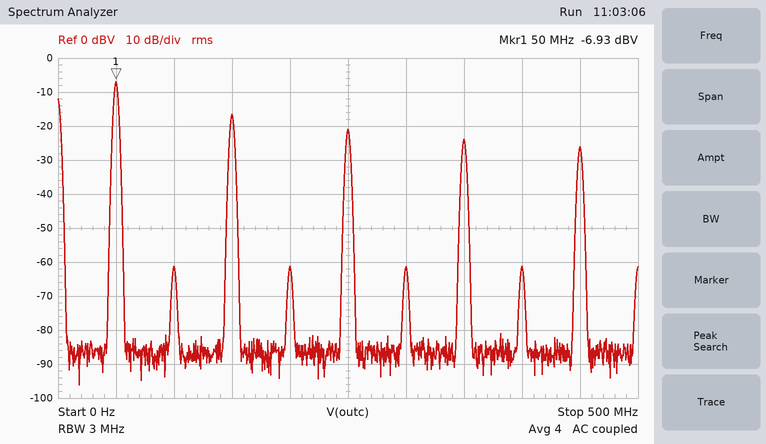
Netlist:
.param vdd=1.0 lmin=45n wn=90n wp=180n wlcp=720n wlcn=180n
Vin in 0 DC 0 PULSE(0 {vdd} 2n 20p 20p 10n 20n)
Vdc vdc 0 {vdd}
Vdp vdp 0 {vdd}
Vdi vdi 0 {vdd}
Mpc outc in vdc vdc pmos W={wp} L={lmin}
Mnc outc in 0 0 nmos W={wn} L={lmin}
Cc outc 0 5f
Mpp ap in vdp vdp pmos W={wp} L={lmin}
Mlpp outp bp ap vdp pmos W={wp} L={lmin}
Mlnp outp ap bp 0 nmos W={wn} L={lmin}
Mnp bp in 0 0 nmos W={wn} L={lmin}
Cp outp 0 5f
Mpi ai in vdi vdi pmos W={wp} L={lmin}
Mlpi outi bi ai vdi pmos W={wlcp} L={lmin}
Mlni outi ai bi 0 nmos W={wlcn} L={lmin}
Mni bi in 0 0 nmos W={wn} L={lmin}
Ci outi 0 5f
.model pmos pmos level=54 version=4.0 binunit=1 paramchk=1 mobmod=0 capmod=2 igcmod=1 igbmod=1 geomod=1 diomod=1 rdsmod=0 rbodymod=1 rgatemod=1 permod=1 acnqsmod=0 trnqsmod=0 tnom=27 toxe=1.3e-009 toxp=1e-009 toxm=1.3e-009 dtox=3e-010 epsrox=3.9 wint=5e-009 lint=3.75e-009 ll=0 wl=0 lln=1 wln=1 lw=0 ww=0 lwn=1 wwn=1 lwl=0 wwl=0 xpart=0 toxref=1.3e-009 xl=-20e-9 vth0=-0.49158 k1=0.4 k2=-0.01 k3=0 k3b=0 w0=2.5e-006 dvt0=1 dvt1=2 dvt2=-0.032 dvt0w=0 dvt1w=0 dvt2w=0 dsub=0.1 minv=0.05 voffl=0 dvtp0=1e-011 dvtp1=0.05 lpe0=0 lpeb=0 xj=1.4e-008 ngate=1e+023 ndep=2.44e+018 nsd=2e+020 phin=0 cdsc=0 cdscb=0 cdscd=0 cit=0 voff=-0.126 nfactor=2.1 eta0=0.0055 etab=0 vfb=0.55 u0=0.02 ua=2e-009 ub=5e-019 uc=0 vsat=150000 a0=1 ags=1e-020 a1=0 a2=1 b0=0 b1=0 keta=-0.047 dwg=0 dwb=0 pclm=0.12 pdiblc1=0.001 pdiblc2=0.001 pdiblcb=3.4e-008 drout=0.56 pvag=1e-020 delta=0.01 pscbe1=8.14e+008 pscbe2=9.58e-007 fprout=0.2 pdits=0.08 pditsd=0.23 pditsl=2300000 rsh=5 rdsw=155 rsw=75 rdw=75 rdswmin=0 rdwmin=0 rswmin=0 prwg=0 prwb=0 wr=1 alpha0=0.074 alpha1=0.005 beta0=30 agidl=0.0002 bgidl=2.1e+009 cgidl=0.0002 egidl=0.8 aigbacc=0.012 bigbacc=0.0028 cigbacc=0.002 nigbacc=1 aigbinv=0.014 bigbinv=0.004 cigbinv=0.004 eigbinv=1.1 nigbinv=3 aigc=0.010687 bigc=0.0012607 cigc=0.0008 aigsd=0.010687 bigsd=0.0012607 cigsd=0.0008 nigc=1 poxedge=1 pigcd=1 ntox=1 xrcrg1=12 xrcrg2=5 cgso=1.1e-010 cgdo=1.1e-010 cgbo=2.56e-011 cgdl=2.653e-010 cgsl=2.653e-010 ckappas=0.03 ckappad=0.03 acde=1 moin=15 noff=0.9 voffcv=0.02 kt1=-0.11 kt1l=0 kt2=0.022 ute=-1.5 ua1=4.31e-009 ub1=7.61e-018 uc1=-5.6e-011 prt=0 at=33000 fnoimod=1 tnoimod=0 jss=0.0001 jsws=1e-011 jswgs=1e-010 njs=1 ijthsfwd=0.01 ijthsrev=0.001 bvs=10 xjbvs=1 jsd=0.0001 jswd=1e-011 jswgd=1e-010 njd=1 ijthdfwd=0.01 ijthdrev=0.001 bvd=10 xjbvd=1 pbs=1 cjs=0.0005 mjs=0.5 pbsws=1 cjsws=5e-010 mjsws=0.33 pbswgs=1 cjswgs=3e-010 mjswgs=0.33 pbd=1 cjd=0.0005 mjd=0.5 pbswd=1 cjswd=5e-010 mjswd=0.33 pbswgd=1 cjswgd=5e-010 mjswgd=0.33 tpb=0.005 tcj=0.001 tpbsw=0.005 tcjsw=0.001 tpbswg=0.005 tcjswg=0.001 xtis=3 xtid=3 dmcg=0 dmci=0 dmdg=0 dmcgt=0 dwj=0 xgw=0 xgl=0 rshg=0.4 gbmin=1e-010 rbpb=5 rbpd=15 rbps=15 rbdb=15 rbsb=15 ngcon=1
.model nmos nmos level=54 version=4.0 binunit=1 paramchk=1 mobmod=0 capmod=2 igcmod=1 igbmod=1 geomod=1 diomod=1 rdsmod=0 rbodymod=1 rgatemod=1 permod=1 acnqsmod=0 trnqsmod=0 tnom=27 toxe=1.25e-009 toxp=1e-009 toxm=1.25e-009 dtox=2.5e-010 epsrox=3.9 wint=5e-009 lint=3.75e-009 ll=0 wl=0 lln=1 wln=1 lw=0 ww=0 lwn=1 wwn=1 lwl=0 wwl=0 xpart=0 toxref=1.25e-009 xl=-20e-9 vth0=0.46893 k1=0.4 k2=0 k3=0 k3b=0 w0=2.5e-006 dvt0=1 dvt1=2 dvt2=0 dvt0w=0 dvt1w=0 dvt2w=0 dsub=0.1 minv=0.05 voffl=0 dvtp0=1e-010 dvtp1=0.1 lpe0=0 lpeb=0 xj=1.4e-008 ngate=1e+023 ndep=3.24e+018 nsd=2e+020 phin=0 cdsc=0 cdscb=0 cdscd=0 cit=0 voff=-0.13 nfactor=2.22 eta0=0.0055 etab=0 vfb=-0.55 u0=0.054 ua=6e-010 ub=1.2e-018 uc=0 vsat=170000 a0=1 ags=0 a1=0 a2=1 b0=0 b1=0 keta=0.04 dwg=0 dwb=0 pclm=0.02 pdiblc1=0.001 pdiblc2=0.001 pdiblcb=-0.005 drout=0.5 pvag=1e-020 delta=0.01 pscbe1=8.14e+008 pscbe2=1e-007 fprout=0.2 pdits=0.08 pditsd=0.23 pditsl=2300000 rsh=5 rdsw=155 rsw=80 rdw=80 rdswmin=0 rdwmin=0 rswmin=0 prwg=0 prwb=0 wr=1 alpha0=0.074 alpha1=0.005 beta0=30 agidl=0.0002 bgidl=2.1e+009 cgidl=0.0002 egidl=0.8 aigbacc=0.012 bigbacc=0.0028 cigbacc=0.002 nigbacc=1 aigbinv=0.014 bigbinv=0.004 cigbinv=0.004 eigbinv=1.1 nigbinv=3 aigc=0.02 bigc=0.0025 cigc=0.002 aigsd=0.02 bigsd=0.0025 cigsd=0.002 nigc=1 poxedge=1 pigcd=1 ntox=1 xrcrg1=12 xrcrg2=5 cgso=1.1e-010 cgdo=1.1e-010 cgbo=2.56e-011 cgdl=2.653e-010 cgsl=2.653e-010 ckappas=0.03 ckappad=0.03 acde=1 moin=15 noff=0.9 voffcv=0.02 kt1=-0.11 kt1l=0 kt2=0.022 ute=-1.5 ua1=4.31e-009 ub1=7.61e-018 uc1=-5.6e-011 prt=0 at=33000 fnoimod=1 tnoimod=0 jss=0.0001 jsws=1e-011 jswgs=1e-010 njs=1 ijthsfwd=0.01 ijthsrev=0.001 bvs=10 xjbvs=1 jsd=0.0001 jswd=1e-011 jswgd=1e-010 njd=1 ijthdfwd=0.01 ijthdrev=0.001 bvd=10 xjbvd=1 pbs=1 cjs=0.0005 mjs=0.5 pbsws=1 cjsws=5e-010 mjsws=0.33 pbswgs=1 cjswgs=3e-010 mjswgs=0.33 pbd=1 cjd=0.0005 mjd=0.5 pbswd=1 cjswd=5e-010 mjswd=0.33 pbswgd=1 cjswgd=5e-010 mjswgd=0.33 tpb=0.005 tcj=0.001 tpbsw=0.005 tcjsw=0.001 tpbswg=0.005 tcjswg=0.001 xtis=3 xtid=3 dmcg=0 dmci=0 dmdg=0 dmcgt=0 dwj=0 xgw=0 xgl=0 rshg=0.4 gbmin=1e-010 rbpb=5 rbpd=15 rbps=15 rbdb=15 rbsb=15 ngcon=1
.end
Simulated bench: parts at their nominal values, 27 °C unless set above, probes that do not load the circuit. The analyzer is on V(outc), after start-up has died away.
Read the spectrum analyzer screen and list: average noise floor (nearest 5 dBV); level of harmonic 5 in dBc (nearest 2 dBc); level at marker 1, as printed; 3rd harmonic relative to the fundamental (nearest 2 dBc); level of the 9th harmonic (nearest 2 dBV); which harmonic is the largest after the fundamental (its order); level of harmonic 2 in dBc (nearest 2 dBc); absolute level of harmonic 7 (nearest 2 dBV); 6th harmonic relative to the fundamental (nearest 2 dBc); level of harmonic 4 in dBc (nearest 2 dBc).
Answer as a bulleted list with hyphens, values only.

- -85 dBV
- -14 dBc
- -6.93 dBV
- -10 dBc
- -26 dBV
- 3
- -54 dBc
- -24 dBV
- -54 dBc
- -54 dBc
